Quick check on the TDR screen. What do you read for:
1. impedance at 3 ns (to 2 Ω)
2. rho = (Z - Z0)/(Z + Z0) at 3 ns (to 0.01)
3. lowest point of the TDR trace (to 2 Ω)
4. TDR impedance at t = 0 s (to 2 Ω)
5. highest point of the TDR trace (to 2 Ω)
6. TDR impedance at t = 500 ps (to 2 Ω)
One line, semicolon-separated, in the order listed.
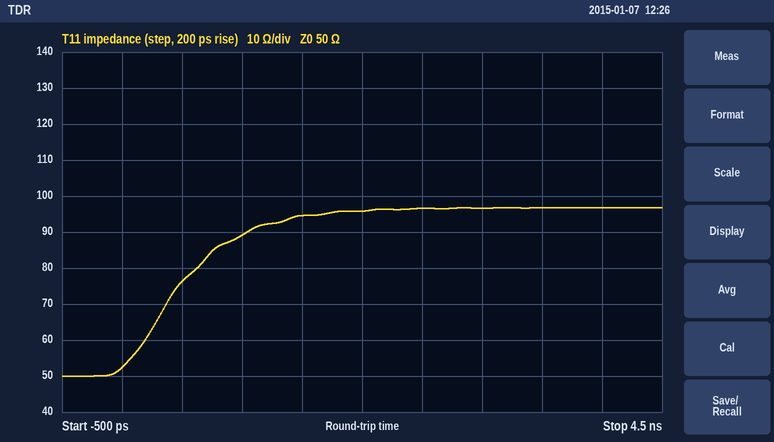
96 Ω; +0.32; 50 Ω; 52 Ω; 96 Ω; 76 Ω
